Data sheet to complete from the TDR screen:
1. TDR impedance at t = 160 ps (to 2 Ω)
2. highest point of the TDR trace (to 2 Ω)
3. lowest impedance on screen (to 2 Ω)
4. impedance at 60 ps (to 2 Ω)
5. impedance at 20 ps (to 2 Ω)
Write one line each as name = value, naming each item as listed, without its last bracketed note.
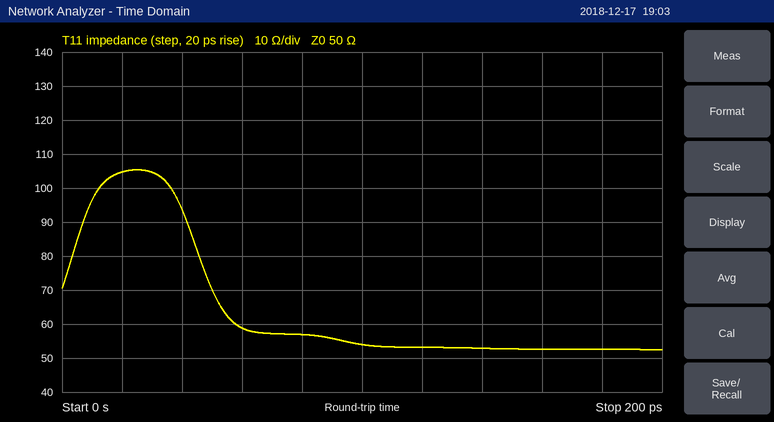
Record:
TDR impedance at t = 160 ps = 52 Ω
highest point of the TDR trace = 106 Ω
lowest impedance on screen = 52 Ω
impedance at 60 ps = 58 Ω
impedance at 20 ps = 104 Ω
